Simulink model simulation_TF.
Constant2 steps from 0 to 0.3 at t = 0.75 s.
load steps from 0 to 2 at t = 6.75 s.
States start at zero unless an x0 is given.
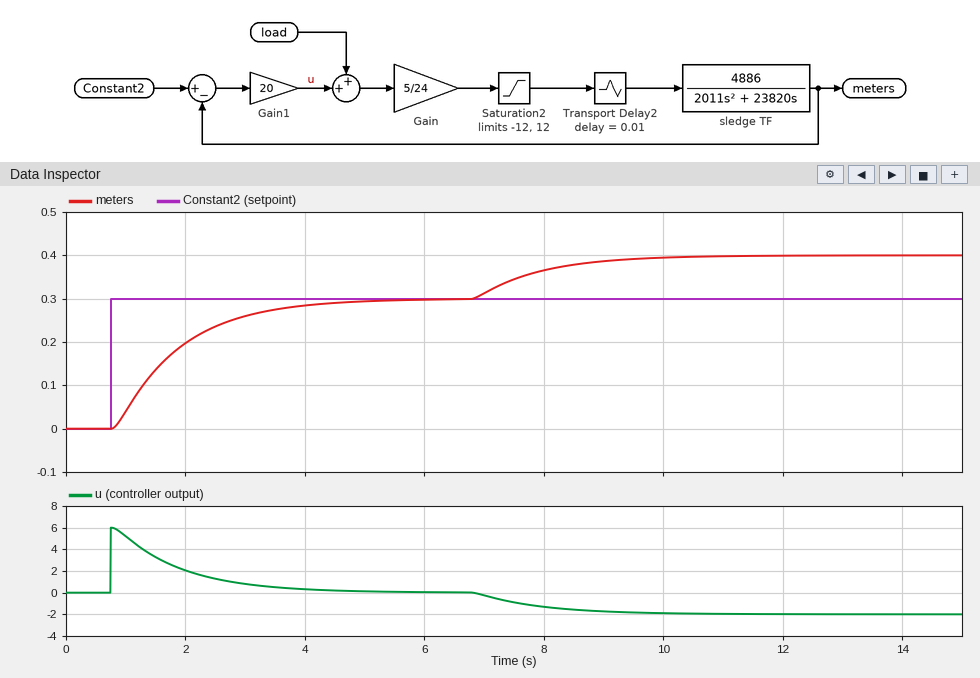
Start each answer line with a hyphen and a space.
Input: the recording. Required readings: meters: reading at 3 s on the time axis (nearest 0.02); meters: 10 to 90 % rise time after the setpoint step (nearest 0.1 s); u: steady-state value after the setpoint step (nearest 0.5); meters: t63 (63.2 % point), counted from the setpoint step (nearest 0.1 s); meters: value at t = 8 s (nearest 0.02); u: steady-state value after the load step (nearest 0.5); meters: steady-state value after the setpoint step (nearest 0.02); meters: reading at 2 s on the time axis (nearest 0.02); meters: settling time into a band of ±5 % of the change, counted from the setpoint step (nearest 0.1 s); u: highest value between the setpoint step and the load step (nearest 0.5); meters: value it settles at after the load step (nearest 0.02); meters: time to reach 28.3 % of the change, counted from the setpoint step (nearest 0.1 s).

- 0.26
- 2.4 s
- 0.0
- 1.2 s
- 0.36
- -2.0
- 0.30
- 0.20
- 3.3 s
- 6.0
- 0.40
- 0.5 s
